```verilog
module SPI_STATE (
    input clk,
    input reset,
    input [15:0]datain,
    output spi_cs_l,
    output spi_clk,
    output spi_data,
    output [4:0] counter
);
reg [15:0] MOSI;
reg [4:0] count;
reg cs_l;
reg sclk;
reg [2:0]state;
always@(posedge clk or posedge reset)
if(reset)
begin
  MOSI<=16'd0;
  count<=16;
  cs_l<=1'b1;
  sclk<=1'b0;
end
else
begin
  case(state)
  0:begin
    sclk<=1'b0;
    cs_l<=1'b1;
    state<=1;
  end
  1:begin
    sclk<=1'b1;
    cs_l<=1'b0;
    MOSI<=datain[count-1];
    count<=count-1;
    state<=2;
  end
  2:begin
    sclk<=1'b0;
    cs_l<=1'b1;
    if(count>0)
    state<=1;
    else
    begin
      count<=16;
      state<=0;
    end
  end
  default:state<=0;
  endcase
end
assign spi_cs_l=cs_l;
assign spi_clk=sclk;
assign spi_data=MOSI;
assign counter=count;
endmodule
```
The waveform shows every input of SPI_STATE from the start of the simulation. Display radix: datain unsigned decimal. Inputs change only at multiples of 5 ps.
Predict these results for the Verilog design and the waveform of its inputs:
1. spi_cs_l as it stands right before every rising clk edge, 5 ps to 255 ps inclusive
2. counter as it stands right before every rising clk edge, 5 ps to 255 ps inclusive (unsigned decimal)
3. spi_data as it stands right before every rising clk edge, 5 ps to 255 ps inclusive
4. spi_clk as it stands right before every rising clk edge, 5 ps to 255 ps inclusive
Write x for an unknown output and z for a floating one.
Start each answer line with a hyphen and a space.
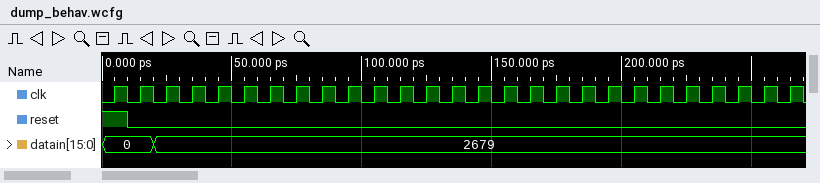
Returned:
- 1 1 1 1 0 1 0 1 0 1 0 1 0 1 0 1 0 1 0 1 0 1 0 1 0 1
- 16, 16, 16, 16, 15, 15, 14, 14, 13, 13, 12, 12, 11, 11, 10, 10, 9, 9, 8, 8, 7, 7, 6, 6, 5, 5
- 0 0 0 0 0 0 0 0 0 0 0 0 1 1 0 0 1 1 0 0 0 0 1 1 1 1
- 0 0 0 0 1 0 1 0 1 0 1 0 1 0 1 0 1 0 1 0 1 0 1 0 1 0
